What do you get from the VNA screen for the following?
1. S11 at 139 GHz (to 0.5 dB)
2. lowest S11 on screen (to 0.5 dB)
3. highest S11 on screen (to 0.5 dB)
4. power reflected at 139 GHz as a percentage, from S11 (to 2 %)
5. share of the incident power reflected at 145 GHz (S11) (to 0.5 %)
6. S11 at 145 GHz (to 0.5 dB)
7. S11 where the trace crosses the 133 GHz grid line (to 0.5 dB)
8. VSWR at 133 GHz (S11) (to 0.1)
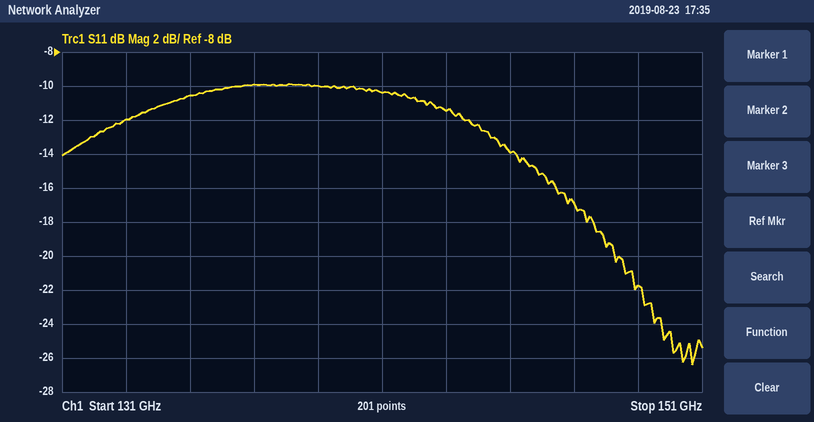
-10.0 dB
-26.5 dB
-10.0 dB
10 %
4.0 %
-14.0 dB
-12.0 dB
1.7
